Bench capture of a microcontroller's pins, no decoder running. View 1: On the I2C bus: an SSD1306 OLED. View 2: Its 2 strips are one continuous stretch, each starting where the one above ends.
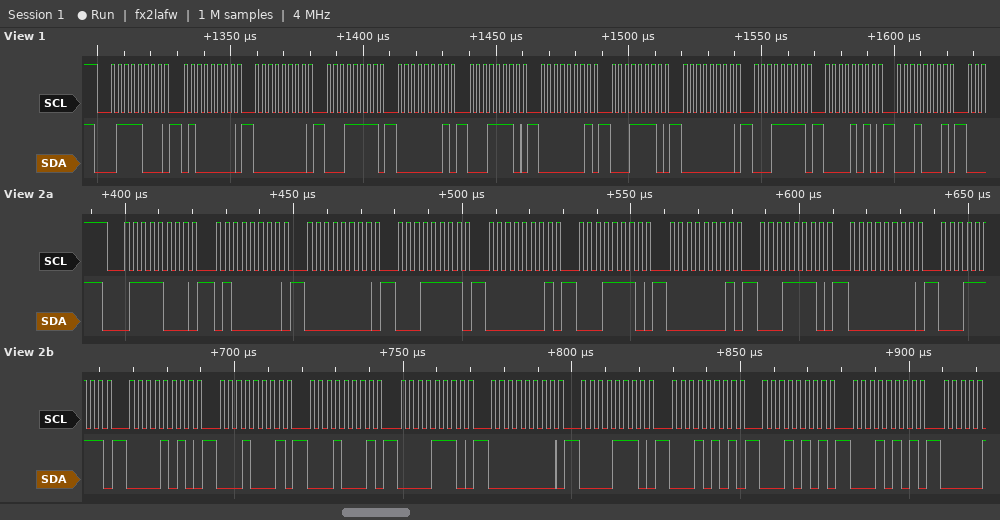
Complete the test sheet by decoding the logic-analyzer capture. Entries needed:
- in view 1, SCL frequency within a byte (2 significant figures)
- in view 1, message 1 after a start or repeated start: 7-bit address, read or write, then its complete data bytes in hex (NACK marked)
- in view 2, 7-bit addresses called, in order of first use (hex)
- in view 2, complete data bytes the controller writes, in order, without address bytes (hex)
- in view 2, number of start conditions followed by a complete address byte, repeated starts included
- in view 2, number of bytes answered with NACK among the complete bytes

400 kHz
0x3C write: 40 00 1F 01 1E 01 1E 00 1F 0A 11
0x3C
40 00 1F 01 1E 01 1E 00 1F 0A 11 11 0E 00 0E 15 15 15
1
0
